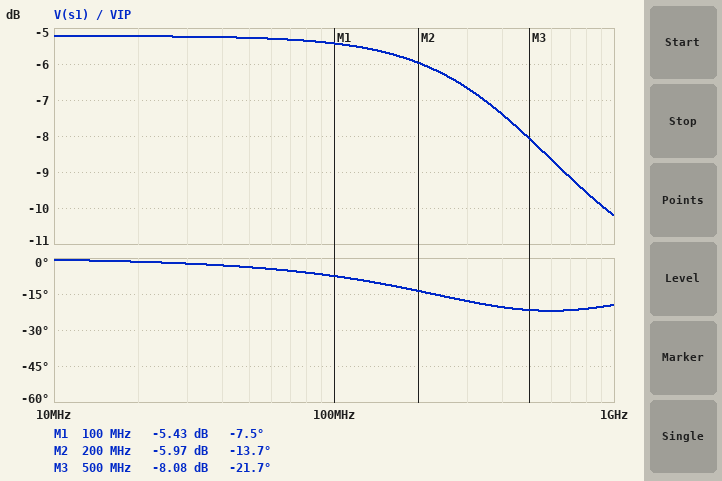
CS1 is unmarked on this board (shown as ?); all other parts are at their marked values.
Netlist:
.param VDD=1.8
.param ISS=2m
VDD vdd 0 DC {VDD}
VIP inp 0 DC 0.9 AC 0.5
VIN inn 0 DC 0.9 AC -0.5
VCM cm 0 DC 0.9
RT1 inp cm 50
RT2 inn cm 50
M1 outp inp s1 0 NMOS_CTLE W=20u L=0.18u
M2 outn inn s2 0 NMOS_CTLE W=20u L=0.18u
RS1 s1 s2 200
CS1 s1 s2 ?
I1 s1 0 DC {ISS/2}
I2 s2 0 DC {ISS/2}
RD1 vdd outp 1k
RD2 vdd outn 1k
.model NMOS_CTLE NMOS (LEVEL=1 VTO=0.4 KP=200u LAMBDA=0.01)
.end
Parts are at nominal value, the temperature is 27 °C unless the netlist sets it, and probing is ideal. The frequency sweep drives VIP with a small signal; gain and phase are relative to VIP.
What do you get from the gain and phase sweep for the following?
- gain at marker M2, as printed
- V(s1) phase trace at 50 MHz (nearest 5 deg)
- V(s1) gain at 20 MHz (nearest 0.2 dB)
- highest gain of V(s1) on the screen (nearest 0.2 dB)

-5.97 dB
-5 deg
-5.2 dB
-5.2 dB
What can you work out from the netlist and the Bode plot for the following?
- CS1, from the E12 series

3.3 pF
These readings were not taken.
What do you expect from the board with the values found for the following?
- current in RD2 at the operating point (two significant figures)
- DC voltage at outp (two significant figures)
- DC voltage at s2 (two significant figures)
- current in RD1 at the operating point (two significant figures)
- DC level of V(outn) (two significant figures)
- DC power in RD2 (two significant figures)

1.0 mA
800 mV
200 mV
1.0 mA
800 mV
1.0 mW
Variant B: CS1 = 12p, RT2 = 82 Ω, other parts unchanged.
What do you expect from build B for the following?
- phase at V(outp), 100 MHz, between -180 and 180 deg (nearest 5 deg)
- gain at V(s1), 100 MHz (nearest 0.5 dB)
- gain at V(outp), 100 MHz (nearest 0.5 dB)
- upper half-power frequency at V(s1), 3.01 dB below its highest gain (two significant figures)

-165 deg
-7.0 dB
12.0 dB
140 MHz
